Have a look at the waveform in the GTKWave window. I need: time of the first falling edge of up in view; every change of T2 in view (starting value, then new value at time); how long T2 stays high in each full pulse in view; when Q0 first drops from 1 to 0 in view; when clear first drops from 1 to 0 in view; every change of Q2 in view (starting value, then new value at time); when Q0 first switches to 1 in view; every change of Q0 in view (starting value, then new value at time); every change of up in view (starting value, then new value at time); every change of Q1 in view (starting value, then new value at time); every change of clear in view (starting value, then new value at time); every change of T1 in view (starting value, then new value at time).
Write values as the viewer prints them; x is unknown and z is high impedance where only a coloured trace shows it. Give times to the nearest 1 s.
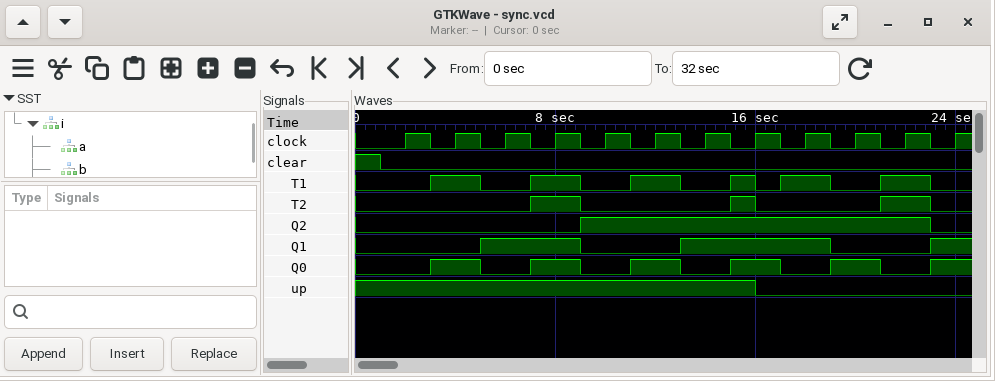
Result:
16 s
0, 1 at 7 s, 0 at 9 s, 1 at 15 s, 0 at 16 s, 1 at 21 s, 0 at 23 s
2 s, 1 s, 2 s
5 s
1 s
0, 1 at 9 s, 0 at 23 s
3 s
0, 1 at 3 s, 0 at 5 s, 1 at 7 s, 0 at 9 s, 1 at 11 s, 0 at 13 s, 1 at 15 s, 0 at 17 s, 1 at 19 s, 0 at 21 s, 1 at 23 s
1, 0 at 16 s
0, 1 at 5 s, 0 at 9 s, 1 at 13 s, 0 at 19 s, 1 at 23 s
1, 0 at 1 s
0, 1 at 3 s, 0 at 5 s, 1 at 7 s, 0 at 9 s, 1 at 11 s, 0 at 13 s, 1 at 15 s, 0 at 16 s, 1 at 17 s, 0 at 19 s, 1 at 21 s, 0 at 23 s
